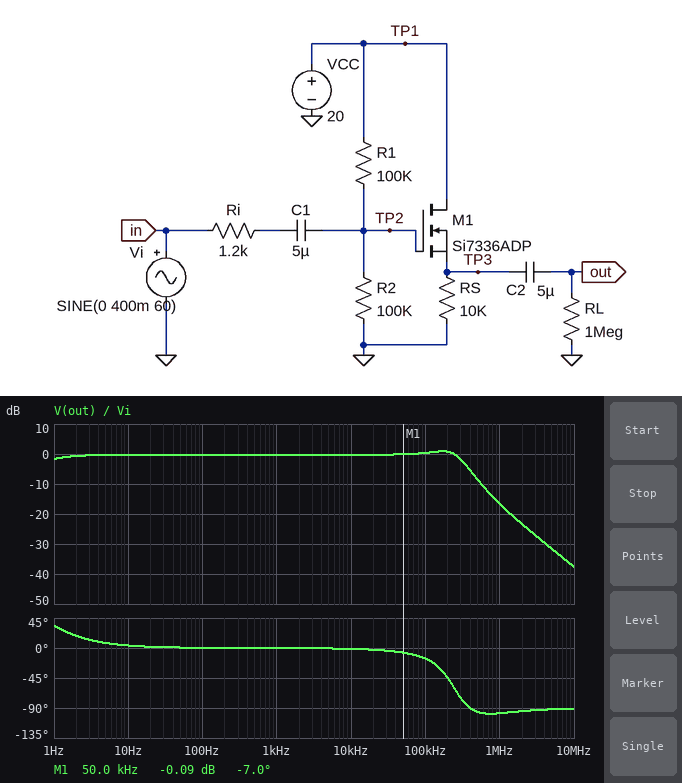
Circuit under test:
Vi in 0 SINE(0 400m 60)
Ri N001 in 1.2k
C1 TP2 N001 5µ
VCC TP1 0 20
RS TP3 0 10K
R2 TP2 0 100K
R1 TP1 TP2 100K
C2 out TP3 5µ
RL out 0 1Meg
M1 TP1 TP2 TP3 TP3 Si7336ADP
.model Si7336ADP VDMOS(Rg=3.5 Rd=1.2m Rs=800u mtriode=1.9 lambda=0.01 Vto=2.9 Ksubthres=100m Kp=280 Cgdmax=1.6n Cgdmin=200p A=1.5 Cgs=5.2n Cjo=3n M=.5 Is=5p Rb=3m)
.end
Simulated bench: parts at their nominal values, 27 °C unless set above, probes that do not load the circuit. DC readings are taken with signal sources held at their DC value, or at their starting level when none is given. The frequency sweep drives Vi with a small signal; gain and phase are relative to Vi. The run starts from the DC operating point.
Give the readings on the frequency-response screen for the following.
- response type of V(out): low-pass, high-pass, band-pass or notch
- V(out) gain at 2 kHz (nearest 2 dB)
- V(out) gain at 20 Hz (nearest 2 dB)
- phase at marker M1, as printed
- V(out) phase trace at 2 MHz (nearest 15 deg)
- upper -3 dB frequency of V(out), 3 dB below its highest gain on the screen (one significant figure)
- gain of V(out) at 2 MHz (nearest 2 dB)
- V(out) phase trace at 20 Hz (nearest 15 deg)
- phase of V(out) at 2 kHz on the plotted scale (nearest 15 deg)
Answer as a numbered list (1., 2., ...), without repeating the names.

1. low-pass
2. 0 dB
3. 0 dB
4. -7.0 deg
5. -90 deg
6. 300 kHz
7. -24 dB
8. 0 deg
9. 0 deg
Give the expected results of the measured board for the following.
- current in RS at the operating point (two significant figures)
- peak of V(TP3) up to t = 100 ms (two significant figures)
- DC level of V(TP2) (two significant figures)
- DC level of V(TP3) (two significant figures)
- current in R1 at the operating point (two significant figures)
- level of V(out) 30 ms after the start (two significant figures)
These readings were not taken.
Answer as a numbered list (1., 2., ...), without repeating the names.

1. 750 µA
2. 7.9 V
3. 10 V
4. 7.5 V
5. 100 µA
6. -370 mV
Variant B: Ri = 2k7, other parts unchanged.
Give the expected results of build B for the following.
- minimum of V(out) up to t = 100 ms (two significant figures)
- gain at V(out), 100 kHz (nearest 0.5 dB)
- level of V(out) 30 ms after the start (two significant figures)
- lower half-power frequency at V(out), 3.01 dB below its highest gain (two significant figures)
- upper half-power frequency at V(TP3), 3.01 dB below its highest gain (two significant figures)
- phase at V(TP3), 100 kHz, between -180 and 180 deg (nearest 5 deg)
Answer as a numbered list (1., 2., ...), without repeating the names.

1. -380 mV
2. 0 dB
3. -360 mV
4. 720 mHz
5. 200 kHz
6. -35 deg
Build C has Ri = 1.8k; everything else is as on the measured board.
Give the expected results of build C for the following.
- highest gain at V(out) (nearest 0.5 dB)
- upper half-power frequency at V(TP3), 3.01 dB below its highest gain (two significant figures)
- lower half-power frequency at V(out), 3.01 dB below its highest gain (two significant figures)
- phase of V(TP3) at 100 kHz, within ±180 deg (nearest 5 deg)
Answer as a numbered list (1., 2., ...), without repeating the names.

1. 0.5 dB
2. 250 kHz
3. 800 mHz
4. -25 deg
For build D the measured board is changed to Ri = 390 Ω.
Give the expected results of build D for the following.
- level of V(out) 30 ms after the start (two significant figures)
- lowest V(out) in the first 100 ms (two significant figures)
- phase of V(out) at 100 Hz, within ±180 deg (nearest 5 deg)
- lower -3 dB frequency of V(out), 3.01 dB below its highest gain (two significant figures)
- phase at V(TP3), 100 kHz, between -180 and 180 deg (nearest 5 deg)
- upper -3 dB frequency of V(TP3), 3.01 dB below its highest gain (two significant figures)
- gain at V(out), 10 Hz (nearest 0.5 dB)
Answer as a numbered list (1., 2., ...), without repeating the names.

1. -380 mV
2. -400 mV
3. 0 deg
4. 800 mHz
5. -5 deg
6. 600 kHz
7. 0 dB
